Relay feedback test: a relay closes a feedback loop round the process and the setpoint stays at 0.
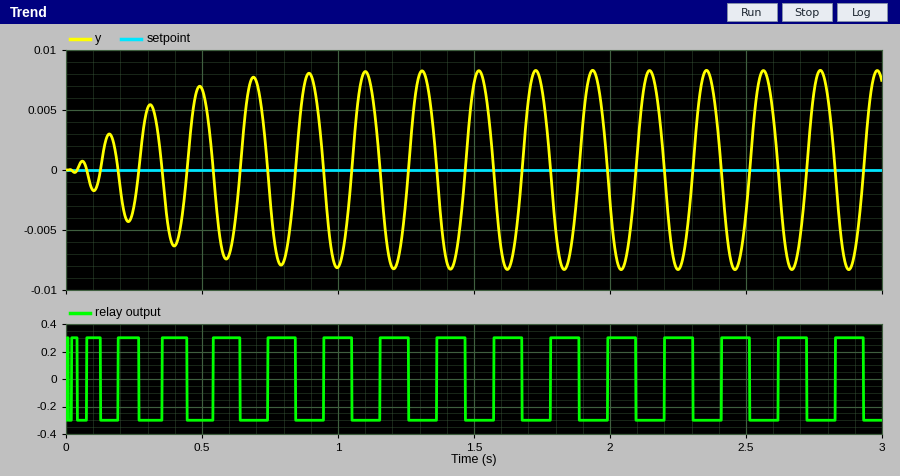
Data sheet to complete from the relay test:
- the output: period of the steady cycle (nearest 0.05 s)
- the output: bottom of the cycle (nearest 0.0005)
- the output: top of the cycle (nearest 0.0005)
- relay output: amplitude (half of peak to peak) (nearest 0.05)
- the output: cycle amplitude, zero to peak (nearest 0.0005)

0.20 s
-0.0085
0.0085
0.30
0.0085
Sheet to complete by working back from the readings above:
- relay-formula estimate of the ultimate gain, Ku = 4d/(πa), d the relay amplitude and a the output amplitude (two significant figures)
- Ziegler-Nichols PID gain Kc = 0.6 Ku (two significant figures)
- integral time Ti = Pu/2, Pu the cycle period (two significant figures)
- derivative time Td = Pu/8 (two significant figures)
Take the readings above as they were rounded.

45
27
0.10 s
0.025 s
